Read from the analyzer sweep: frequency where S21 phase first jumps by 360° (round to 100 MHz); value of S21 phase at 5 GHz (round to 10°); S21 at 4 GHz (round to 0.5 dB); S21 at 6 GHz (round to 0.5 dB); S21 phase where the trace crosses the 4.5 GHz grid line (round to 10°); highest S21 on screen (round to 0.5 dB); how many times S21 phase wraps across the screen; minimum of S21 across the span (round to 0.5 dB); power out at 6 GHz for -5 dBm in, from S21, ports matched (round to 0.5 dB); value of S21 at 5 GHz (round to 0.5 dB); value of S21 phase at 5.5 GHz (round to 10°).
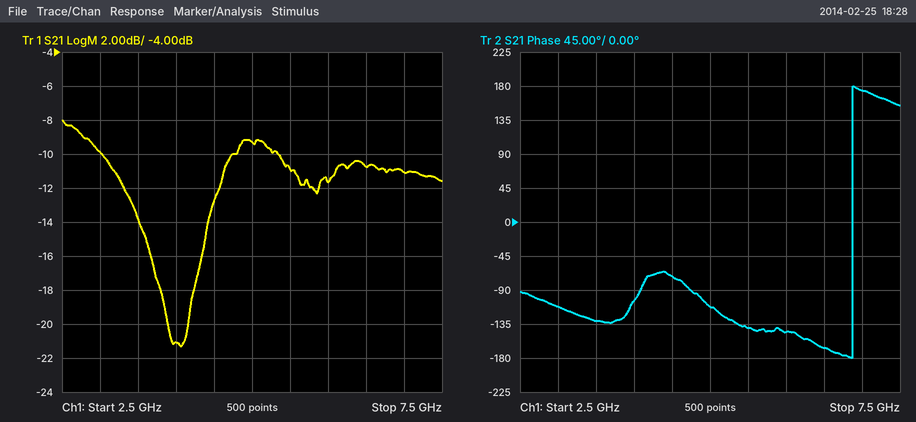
6.9 GHz
-110°
-21.0 dB
-11.5 dB
-70°
-8.0 dB
1
-21.5 dB
-16.5 dBm
-9.5 dB
-140°
